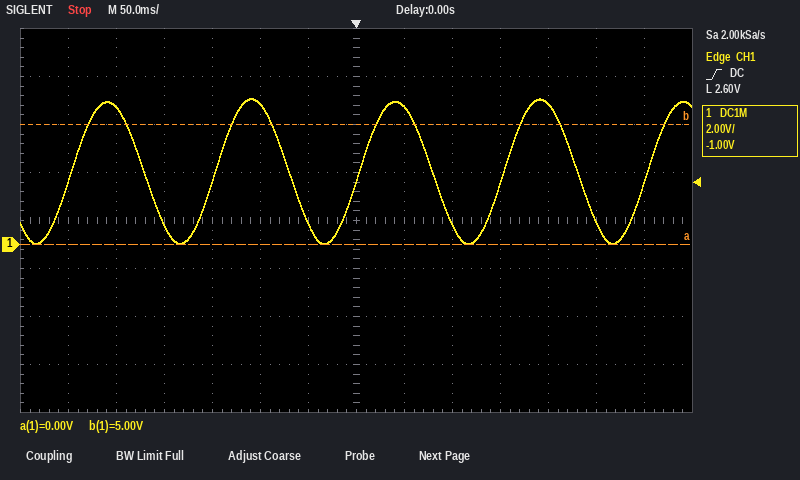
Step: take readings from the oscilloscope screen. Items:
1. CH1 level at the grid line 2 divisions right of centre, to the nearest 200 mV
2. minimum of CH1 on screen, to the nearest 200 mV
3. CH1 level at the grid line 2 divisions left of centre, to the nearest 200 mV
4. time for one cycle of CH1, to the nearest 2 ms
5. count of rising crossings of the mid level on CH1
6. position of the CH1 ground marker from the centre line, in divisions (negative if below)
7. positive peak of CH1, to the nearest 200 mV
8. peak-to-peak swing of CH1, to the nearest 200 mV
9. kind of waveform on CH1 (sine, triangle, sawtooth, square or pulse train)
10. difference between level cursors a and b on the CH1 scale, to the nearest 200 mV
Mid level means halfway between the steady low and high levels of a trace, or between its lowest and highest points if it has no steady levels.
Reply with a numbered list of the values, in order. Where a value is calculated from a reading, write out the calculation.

1. 800 mV
2. 0.0 V
3. 5.8 V
4. 150 ms
5. 5
6. -0.5 div
7. 6.0 V
8. 6.0 V − (0.0 V) = 6.0 V
9. sine
10. 5.0 V
